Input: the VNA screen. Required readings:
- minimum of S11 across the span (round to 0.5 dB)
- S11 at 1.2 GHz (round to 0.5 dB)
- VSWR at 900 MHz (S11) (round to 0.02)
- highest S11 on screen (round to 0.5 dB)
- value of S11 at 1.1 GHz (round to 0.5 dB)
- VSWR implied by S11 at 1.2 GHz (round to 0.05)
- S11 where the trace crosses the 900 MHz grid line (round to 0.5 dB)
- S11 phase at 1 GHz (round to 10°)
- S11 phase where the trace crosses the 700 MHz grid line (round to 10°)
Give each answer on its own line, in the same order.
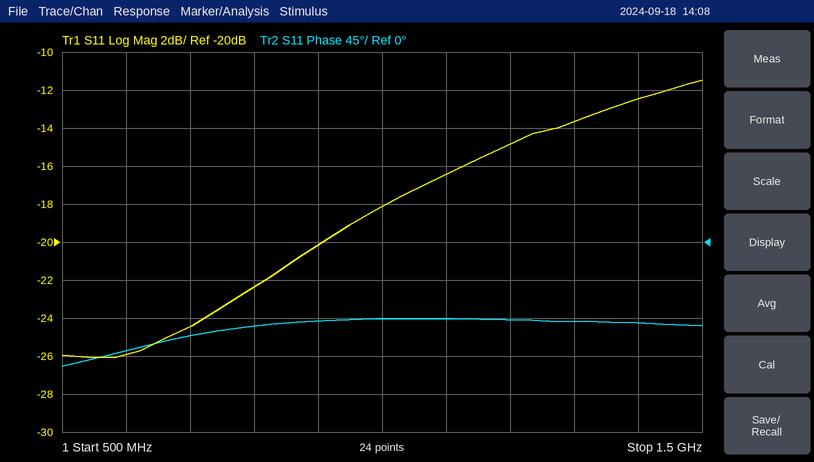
-26.0 dB
-15.0 dB
1.22
-11.5 dB
-16.5 dB
1.45
-20.0 dB
-90°
-110°
